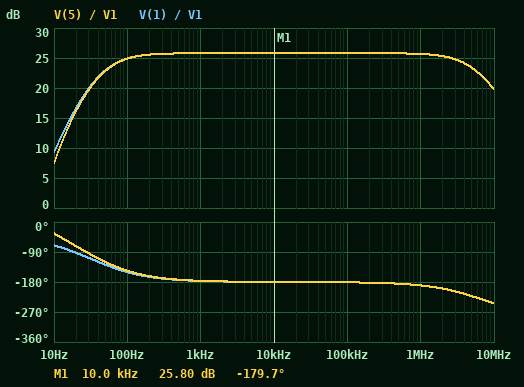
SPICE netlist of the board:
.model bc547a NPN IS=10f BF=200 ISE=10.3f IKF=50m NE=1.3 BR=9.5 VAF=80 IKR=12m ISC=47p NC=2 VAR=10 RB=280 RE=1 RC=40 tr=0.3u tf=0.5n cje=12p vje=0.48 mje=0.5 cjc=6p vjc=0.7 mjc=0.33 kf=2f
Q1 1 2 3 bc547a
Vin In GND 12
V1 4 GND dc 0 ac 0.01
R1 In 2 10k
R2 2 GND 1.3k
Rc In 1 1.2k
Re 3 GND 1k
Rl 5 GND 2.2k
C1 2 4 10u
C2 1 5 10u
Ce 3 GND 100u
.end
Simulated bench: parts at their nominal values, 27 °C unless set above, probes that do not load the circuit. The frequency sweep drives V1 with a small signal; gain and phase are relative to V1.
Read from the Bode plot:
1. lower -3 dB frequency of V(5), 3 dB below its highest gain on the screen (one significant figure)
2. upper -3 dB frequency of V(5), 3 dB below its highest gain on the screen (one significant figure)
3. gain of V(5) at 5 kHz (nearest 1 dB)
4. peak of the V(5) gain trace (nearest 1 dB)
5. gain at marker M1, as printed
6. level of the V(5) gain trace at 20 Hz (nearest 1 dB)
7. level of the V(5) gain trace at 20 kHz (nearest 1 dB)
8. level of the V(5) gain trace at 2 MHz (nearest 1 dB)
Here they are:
50 Hz
6 MHz
26 dB
26 dB
25.80 dB
16 dB
26 dB
25 dB
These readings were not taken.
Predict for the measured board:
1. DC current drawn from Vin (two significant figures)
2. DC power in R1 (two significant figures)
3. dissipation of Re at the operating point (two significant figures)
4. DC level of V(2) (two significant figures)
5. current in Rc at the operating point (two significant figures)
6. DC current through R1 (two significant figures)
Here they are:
1.8 mA
11 mW
530 µW
1.4 V
720 µA
1.1 mA
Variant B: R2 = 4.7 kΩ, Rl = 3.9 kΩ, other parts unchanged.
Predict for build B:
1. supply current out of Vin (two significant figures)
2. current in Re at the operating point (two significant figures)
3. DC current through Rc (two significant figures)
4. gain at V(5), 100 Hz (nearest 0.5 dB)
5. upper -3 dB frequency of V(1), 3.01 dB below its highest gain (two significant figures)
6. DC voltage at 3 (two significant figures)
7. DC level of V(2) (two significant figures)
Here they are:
3.9 mA
3.1 mA
3.0 mA
32.5 dB
1.8 MHz
3.1 V
3.8 V
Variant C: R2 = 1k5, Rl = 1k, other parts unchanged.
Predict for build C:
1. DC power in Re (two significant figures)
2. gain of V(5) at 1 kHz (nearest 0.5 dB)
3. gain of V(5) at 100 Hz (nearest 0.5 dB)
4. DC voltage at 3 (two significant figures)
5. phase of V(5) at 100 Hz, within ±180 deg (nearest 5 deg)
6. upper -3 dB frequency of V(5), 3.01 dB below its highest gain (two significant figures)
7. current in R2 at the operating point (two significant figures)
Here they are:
810 µW
24.5 dB
23.0 dB
900 mV
-140 deg
6.1 MHz
1.0 mA
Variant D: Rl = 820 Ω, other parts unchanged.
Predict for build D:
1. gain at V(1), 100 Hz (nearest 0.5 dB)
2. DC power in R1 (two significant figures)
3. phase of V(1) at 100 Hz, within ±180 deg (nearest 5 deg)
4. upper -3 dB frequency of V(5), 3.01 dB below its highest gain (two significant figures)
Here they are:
21.0 dB
11 mW
-155 deg
7.2 MHz
